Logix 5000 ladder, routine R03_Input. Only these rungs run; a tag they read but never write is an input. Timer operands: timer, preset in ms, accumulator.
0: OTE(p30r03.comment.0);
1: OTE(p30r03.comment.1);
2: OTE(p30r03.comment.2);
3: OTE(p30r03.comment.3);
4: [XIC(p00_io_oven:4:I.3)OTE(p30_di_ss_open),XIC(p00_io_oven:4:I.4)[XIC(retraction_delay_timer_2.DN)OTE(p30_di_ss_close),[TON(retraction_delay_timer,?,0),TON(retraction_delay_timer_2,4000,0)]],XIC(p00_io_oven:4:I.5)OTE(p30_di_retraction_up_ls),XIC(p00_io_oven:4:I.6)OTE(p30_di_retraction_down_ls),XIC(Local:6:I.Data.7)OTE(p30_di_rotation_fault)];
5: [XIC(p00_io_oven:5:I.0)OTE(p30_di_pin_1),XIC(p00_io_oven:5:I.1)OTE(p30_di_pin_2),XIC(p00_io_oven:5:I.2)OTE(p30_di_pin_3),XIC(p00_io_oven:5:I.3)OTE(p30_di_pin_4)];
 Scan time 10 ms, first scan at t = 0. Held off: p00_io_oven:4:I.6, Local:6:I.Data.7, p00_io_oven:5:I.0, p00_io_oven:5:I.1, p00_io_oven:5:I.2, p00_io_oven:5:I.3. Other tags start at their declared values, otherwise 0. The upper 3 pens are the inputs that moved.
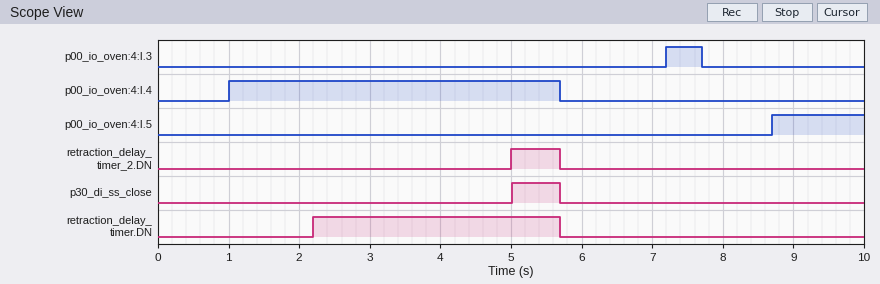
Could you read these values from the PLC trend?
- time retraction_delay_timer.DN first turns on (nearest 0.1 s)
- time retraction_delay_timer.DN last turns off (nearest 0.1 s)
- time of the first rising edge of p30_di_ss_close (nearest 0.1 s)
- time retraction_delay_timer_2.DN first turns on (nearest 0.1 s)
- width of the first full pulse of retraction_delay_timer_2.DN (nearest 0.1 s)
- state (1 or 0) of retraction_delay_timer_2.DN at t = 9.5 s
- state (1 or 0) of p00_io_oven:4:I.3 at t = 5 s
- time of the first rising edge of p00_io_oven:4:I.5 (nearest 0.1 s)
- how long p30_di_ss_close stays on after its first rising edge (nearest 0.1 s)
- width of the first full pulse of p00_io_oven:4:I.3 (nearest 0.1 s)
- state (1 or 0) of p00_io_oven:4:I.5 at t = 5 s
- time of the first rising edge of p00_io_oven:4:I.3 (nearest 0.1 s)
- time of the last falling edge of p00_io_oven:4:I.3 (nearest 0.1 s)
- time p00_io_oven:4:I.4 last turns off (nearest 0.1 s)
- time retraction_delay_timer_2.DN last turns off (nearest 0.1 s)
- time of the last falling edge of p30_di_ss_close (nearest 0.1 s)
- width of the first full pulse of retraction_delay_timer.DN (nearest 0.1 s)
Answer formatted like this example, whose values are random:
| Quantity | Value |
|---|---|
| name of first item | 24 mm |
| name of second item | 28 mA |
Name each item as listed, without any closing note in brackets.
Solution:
| Quantity | Value |
|---|---|
| time retraction_delay_timer.DN first turns on | 2.2 s |
| time retraction_delay_timer.DN last turns off | 5.7 s |
| time of the first rising edge of p30_di_ss_close | 5.0 s |
| time retraction_delay_timer_2.DN first turns on | 5.0 s |
| width of the first full pulse of retraction_delay_timer_2.DN | 0.7 s |
| state (1 or 0) of retraction_delay_timer_2.DN at t = 9.5 s | 0 |
| state (1 or 0) of p00_io_oven:4:I.3 at t = 5 s | 0 |
| time of the first rising edge of p00_io_oven:4:I.5 | 8.7 s |
| how long p30_di_ss_close stays on after its first rising edge | 0.7 s |
| width of the first full pulse of p00_io_oven:4:I.3 | 0.5 s |
| state (1 or 0) of p00_io_oven:4:I.5 at t = 5 s | 0 |
| time of the first rising edge of p00_io_oven:4:I.3 | 7.2 s |
| time of the last falling edge of p00_io_oven:4:I.3 | 7.7 s |
| time p00_io_oven:4:I.4 last turns off | 5.7 s |
| time retraction_delay_timer_2.DN last turns off | 5.7 s |
| time of the last falling edge of p30_di_ss_close | 5.7 s |
| width of the first full pulse of retraction_delay_timer.DN | 3.5 s |
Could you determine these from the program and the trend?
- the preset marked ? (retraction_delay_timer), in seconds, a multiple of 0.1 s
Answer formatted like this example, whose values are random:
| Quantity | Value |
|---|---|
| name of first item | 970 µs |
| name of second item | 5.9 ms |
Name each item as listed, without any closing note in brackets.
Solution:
| Quantity | Value |
|---|---|
| the preset marked ? (retraction_delay_timer), in seconds, a multiple of 0.1 s | 1.2 s |
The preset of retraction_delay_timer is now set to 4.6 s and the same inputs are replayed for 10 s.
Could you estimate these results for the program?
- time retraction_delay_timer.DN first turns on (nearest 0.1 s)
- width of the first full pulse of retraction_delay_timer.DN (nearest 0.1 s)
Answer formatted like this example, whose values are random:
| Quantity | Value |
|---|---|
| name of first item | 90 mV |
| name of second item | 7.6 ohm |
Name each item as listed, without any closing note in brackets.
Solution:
| Quantity | Value |
|---|---|
| time retraction_delay_timer.DN first turns on | 5.6 s |
| width of the first full pulse of retraction_delay_timer.DN | 0.1 s |
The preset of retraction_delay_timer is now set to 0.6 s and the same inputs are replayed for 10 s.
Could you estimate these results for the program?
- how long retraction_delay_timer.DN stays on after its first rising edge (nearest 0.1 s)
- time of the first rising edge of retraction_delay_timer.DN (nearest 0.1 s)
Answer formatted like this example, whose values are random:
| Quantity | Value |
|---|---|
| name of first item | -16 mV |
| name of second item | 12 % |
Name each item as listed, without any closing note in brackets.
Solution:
| Quantity | Value |
|---|---|
| how long retraction_delay_timer.DN stays on after its first rising edge | 4.1 s |
| time of the first rising edge of retraction_delay_timer.DN | 1.6 s |
